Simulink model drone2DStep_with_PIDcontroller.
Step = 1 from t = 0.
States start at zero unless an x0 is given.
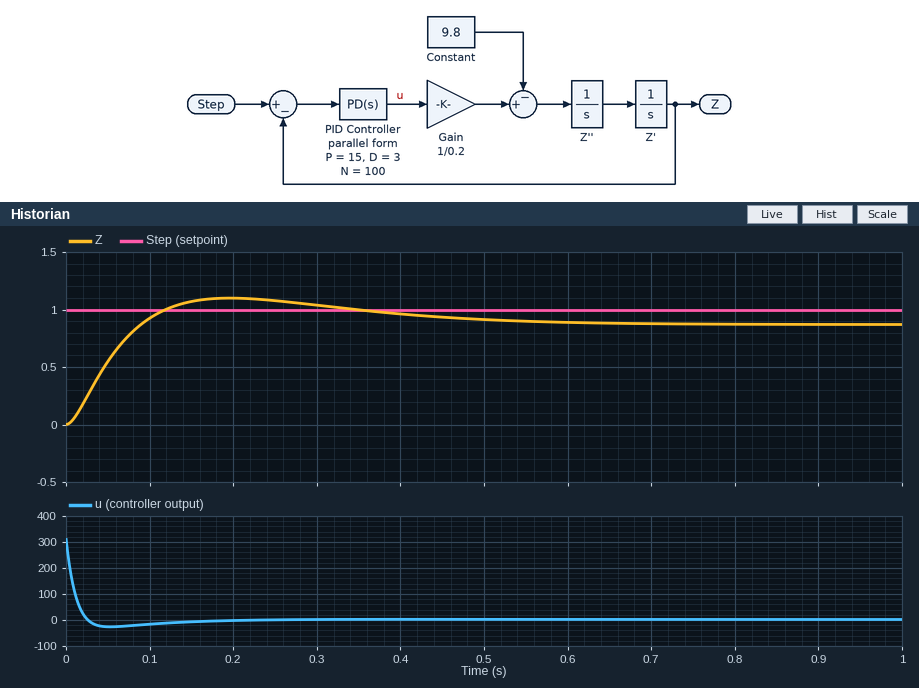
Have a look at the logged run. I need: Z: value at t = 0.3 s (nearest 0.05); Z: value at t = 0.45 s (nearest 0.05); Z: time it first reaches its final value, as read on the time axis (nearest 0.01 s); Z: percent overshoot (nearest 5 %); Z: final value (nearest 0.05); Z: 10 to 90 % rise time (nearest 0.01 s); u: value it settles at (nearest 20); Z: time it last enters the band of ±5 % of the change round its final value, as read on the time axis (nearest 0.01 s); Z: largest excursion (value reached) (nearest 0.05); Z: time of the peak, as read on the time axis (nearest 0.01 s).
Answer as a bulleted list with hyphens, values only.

- 1.05
- 0.95
- 0.09 s
- 25 %
- 0.85
- 0.06 s
- 0
- 0.50 s
- 1.10
- 0.20 s
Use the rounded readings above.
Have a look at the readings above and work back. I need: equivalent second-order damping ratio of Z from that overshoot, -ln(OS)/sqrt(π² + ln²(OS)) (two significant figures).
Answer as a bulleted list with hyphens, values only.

- 0.40
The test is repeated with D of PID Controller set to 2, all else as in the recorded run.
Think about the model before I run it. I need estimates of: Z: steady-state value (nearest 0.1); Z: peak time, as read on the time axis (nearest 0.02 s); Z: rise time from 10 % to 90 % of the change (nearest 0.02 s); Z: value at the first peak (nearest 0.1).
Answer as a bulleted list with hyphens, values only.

- 0.9
- 0.24 s
- 0.08 s
- 1.2
